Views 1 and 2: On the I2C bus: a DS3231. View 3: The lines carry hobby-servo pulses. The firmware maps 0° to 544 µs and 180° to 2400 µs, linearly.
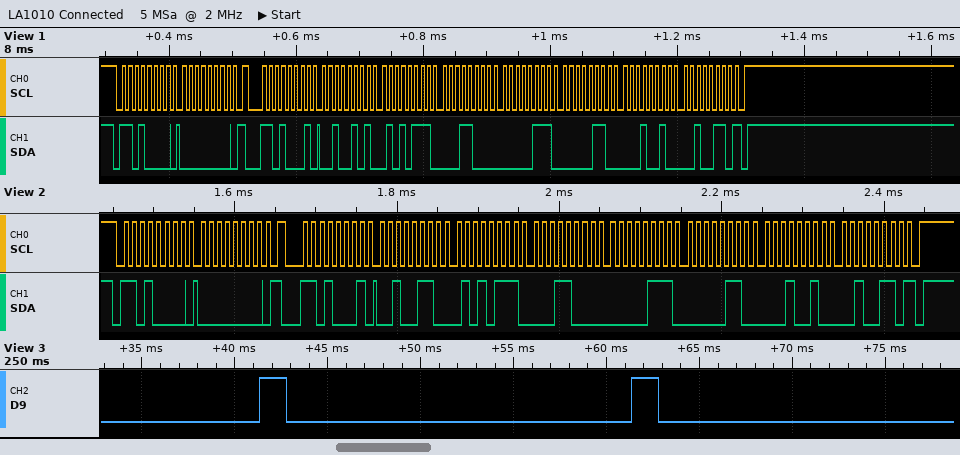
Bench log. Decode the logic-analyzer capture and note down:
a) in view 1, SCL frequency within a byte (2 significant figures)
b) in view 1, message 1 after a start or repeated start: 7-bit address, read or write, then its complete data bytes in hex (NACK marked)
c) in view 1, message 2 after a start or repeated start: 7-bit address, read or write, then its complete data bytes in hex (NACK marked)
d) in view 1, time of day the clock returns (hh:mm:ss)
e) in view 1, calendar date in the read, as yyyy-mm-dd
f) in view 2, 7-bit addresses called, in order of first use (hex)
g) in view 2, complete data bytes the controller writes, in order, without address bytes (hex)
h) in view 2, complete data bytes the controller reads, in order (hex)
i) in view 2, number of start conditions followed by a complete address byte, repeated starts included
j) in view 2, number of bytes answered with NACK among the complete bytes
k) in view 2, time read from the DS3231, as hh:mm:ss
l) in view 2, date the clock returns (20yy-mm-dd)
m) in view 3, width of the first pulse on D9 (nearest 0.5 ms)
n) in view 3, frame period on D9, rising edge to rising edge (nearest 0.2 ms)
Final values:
100 kHz
0x68 write: 00
0x68 read: 25 57 18 07 06 12 26 NACK
18:57:25
2026-12-06
0x68
00
26 57 18 07 06 12 26
2
1
18:57:26
2026-12-06
1.5 ms
20.0 ms
